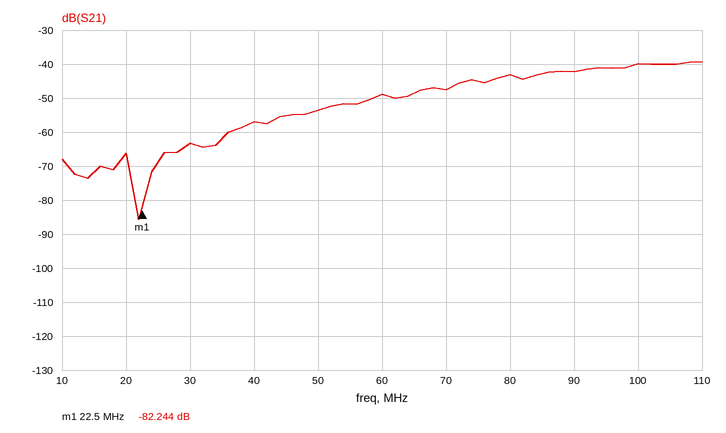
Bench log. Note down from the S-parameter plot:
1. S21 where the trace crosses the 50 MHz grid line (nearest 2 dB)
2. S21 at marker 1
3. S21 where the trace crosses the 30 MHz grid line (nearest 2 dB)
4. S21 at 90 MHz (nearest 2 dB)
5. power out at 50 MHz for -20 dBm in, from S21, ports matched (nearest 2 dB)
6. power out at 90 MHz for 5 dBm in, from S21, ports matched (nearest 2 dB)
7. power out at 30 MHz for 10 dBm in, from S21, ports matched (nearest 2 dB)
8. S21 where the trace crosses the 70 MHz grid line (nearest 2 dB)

-54 dB
-82.244 dB
-64 dB
-42 dB
-74 dBm
-38 dBm
-54 dBm
-48 dB
